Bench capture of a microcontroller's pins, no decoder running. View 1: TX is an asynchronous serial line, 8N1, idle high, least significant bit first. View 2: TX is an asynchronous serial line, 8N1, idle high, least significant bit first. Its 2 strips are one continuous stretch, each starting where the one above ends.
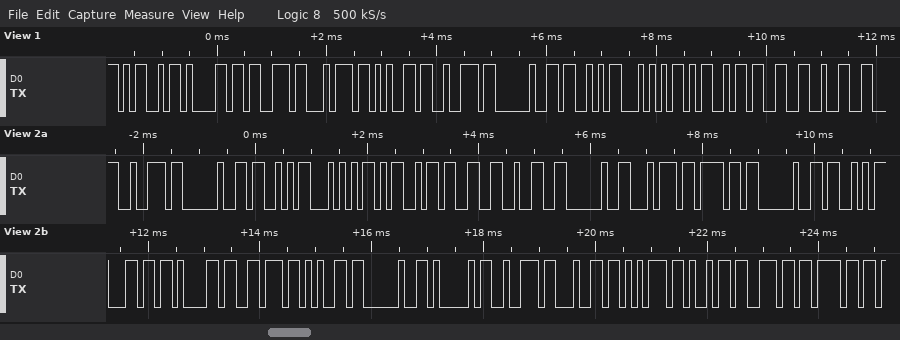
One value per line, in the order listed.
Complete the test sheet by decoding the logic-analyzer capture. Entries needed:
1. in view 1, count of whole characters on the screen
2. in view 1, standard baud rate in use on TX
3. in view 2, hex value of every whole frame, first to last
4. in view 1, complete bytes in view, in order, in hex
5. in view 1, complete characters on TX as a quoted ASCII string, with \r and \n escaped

12
9600 baud
0x72 0x20 0x53 0x54 0x4D 0x33 0x32 0x20 0x74 0x6F 0x20 0x53 0x6C 0x61 0x76 0x65 0x20 0x41 0x72 0x64 0x75 0x69 0x6E 0x6F
4D 61 73 74 65 72 20 53 54 4D 33 32
"Master STM32"
